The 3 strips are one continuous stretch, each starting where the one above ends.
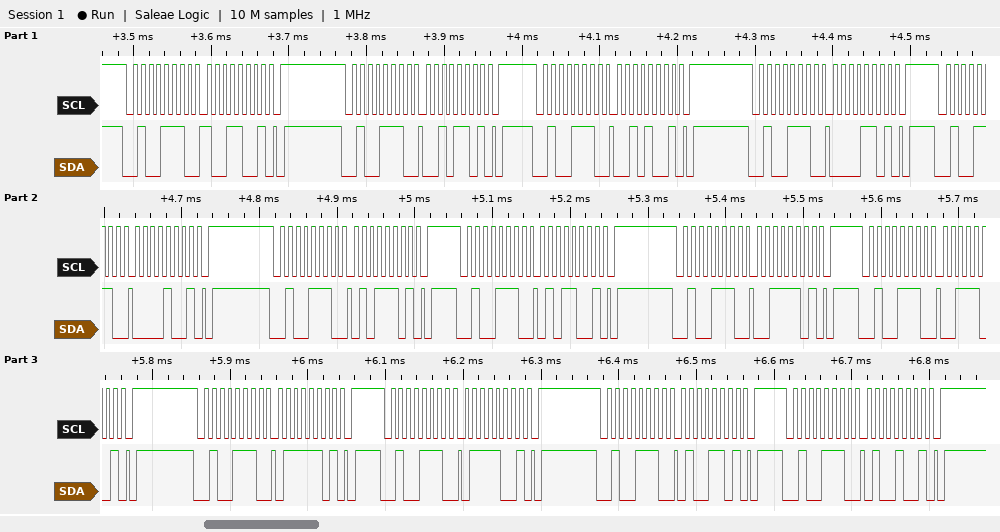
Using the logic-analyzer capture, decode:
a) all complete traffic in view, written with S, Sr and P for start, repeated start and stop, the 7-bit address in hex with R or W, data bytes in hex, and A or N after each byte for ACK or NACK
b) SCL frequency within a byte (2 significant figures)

S 27W A 99 A P S 27W A 2D A P S 27W A 29 A P S 27W A 0D A P S 27W A 09 A P S 27W A 5D A P S 27W A 59 A P S 27W A 3D A P S 27W A 39 A P S 27W A 7D A P S 27W A 79 A P S 27W A 4D A P S 27W A 49 A P
100 kHz
